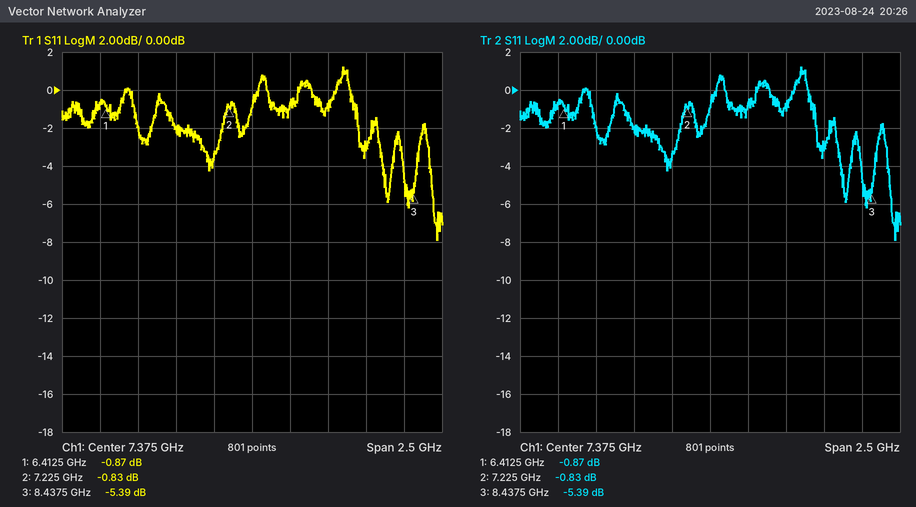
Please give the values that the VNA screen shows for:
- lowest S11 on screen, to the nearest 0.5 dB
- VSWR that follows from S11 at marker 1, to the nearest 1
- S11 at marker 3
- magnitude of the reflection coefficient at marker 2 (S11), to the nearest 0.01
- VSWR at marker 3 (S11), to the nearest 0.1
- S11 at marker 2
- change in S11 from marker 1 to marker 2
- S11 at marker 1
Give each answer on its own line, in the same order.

-8.0 dB
20
-5.39 dB
0.91
3.3
-0.83 dB
0.04 dB
-0.87 dB
